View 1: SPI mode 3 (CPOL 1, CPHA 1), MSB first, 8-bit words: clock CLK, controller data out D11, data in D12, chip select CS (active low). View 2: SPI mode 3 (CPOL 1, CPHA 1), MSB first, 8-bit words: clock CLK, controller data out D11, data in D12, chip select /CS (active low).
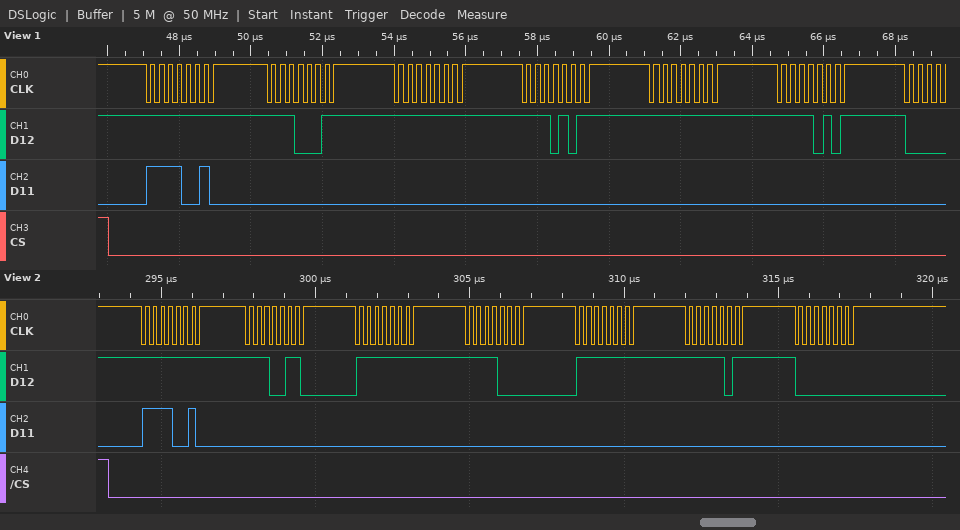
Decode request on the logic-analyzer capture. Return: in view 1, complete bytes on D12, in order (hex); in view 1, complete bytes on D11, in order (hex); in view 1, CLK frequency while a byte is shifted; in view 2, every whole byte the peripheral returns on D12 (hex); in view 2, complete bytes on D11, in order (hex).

FF E3 FF EB FF F5
F2 00 00 00 00 00
4 MHz
0xFF 0xE6 0xFF 0xF0 0xFF 0xFB 0x00
0xF2 0x00 0x00 0x00 0x00 0x00 0x00
